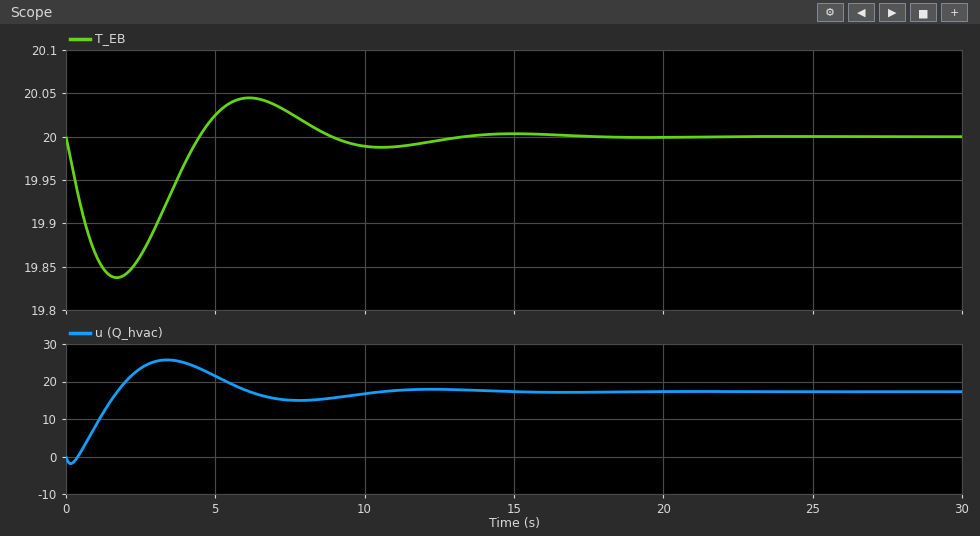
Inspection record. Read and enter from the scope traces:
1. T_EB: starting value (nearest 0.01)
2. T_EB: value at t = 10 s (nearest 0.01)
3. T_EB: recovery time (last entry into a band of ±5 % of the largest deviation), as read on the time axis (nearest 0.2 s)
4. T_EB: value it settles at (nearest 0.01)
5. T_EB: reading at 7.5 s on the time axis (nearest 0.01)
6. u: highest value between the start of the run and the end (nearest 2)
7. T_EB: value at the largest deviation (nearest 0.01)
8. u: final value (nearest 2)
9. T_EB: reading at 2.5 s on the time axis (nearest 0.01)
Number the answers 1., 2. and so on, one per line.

1. 20.00
2. 19.99
3. 11.8 s
4. 20.00
5. 20.03
6. 26
7. 19.84
8. 18
9. 19.86
